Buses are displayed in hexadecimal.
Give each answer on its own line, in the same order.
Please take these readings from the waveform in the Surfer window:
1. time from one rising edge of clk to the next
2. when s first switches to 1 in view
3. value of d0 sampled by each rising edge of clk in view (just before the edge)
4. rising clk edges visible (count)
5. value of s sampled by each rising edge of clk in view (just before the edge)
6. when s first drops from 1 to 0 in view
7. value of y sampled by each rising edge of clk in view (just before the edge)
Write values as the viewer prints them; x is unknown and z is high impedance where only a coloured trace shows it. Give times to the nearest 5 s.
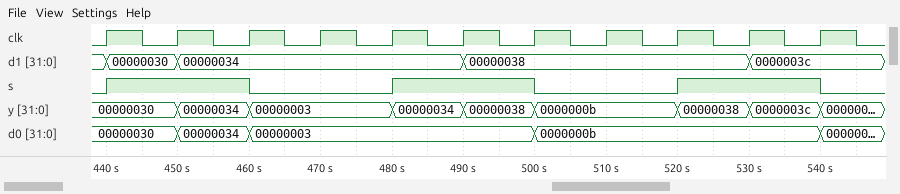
10 s
440 s
00000030, 00000030, 00000034, 00000003, 00000003, 00000003, 00000003, 0000000b, 0000000b, 0000000b, 0000000b
11
0 1 1 0 0 1 1 0 0 1 1
460 s
00000030, 00000030, 00000034, 00000003, 00000003, 00000034, 00000038, 0000000b, 0000000b, 00000038, 0000003c
